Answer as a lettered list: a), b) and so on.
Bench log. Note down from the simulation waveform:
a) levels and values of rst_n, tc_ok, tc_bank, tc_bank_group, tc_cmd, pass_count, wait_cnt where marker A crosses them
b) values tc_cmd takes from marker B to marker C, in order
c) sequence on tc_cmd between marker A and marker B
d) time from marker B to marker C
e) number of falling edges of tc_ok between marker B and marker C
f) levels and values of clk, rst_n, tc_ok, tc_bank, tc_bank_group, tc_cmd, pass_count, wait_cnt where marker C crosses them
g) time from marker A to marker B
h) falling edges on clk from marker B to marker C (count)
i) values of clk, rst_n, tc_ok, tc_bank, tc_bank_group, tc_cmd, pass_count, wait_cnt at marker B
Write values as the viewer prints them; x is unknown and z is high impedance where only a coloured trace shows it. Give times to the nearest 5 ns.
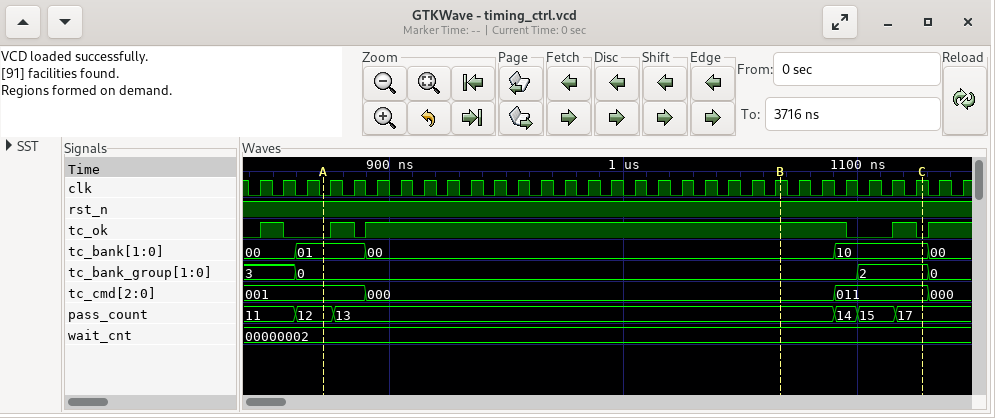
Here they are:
a) rst_n=1, tc_ok=0, tc_bank=01, tc_bank_group=0, tc_cmd=001, pass_count=12, wait_cnt=00000002
b) 000, 011
c) 001, 000
d) 60 ns
e) 2
f) clk=1, rst_n=1, tc_ok=0, tc_bank=10, tc_bank_group=2, tc_cmd=011, pass_count=17, wait_cnt=00000002
g) 195 ns
h) 6
i) clk=1, rst_n=1, tc_ok=1, tc_bank=00, tc_bank_group=0, tc_cmd=000, pass_count=13, wait_cnt=00000002
